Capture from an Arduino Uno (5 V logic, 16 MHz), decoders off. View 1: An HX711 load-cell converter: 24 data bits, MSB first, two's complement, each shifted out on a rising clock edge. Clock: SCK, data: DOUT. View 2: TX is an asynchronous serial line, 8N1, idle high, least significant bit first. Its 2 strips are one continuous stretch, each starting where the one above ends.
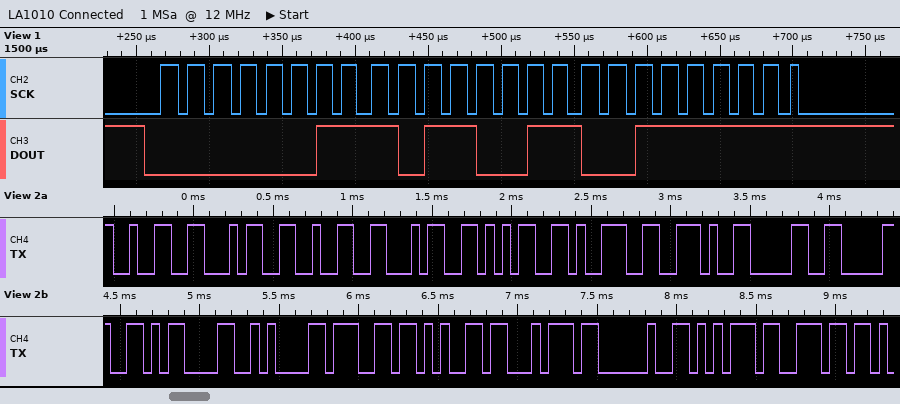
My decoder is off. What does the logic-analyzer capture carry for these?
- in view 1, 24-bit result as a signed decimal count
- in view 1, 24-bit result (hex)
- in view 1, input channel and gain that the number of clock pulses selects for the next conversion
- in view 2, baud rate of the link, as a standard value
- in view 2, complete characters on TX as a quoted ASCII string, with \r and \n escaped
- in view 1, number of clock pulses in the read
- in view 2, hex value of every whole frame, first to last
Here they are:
242495
0x03B33F
channel A, gain 128
19200 baud
"242459.00\r\nget un"
25
32 34 32 34 35 39 2E 30 30 0D 0A 67 65 74 20 75 6E
